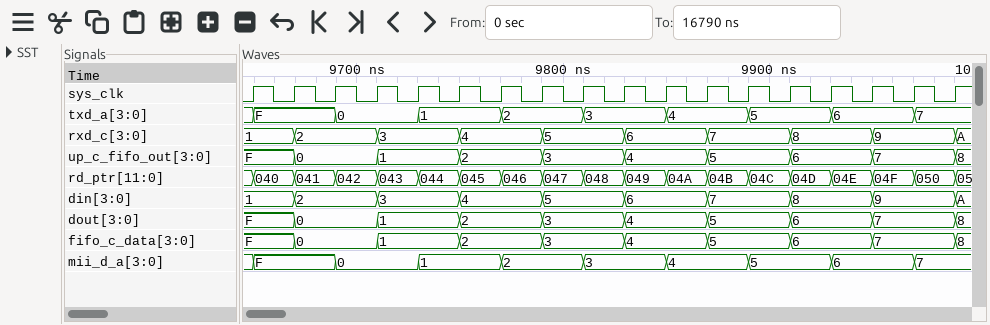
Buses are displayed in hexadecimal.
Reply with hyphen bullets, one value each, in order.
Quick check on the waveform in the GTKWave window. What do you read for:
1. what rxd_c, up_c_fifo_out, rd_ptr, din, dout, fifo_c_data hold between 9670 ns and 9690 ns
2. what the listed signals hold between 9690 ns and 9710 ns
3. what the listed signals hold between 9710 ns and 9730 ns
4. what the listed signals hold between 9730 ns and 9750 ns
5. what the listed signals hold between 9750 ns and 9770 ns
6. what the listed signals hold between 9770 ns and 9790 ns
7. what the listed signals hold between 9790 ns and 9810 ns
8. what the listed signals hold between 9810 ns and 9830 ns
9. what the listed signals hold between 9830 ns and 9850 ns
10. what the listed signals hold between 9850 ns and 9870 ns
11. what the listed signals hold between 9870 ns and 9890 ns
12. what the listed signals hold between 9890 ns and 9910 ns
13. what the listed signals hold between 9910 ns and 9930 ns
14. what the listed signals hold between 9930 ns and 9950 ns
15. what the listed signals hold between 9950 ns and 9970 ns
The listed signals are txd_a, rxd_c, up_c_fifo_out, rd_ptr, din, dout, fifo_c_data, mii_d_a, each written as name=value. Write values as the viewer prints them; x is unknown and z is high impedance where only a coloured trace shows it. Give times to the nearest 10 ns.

- rxd_c=2, up_c_fifo_out=0, rd_ptr=041, din=2, dout=0, fifo_c_data=0
- txd_a=0, rxd_c=2, up_c_fifo_out=0, rd_ptr=042, din=2, dout=0, fifo_c_data=0, mii_d_a=0
- txd_a=0, rxd_c=3, up_c_fifo_out=1, rd_ptr=043, din=3, dout=1, fifo_c_data=1, mii_d_a=0
- txd_a=1, rxd_c=3, up_c_fifo_out=1, rd_ptr=044, din=3, dout=1, fifo_c_data=1, mii_d_a=1
- txd_a=1, rxd_c=4, up_c_fifo_out=2, rd_ptr=045, din=4, dout=2, fifo_c_data=2, mii_d_a=1
- txd_a=2, rxd_c=4, up_c_fifo_out=2, rd_ptr=046, din=4, dout=2, fifo_c_data=2, mii_d_a=2
- txd_a=2, rxd_c=5, up_c_fifo_out=3, rd_ptr=047, din=5, dout=3, fifo_c_data=3, mii_d_a=2
- txd_a=3, rxd_c=5, up_c_fifo_out=3, rd_ptr=048, din=5, dout=3, fifo_c_data=3, mii_d_a=3
- txd_a=3, rxd_c=6, up_c_fifo_out=4, rd_ptr=049, din=6, dout=4, fifo_c_data=4, mii_d_a=3
- txd_a=4, rxd_c=6, up_c_fifo_out=4, rd_ptr=04A, din=6, dout=4, fifo_c_data=4, mii_d_a=4
- txd_a=4, rxd_c=7, up_c_fifo_out=5, rd_ptr=04B, din=7, dout=5, fifo_c_data=5, mii_d_a=4
- txd_a=5, rxd_c=7, up_c_fifo_out=5, rd_ptr=04C, din=7, dout=5, fifo_c_data=5, mii_d_a=5
- txd_a=5, rxd_c=8, up_c_fifo_out=6, rd_ptr=04D, din=8, dout=6, fifo_c_data=6, mii_d_a=5
- txd_a=6, rxd_c=8, up_c_fifo_out=6, rd_ptr=04E, din=8, dout=6, fifo_c_data=6, mii_d_a=6
- txd_a=6, rxd_c=9, up_c_fifo_out=7, rd_ptr=04F, din=9, dout=7, fifo_c_data=7, mii_d_a=6
